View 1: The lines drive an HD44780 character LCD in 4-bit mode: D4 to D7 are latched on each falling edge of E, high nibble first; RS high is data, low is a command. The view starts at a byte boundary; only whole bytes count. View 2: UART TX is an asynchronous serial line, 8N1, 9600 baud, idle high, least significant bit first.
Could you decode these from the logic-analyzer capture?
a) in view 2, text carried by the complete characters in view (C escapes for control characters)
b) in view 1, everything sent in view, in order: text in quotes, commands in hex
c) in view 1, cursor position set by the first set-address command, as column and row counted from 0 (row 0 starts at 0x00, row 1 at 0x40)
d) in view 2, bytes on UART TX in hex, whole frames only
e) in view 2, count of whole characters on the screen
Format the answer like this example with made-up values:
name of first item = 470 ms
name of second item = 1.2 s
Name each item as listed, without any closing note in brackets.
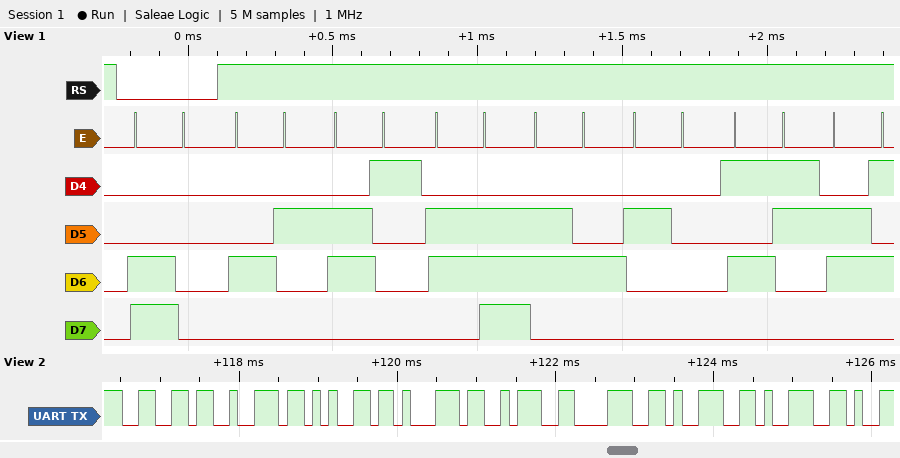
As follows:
in view 2, text carried by the complete characters in view = "freq:899"
in view 1, everything sent in view, in order: text in quotes, commands in hex = 0xC0 "Band Se"
in view 1, cursor position set by the first set-address command, as column and row counted from 0 = column 0, row 1
in view 2, bytes on UART TX in hex, whole frames only = 66 72 65 71 3A 38 39 39
in view 2, count of whole characters on the screen = 8
